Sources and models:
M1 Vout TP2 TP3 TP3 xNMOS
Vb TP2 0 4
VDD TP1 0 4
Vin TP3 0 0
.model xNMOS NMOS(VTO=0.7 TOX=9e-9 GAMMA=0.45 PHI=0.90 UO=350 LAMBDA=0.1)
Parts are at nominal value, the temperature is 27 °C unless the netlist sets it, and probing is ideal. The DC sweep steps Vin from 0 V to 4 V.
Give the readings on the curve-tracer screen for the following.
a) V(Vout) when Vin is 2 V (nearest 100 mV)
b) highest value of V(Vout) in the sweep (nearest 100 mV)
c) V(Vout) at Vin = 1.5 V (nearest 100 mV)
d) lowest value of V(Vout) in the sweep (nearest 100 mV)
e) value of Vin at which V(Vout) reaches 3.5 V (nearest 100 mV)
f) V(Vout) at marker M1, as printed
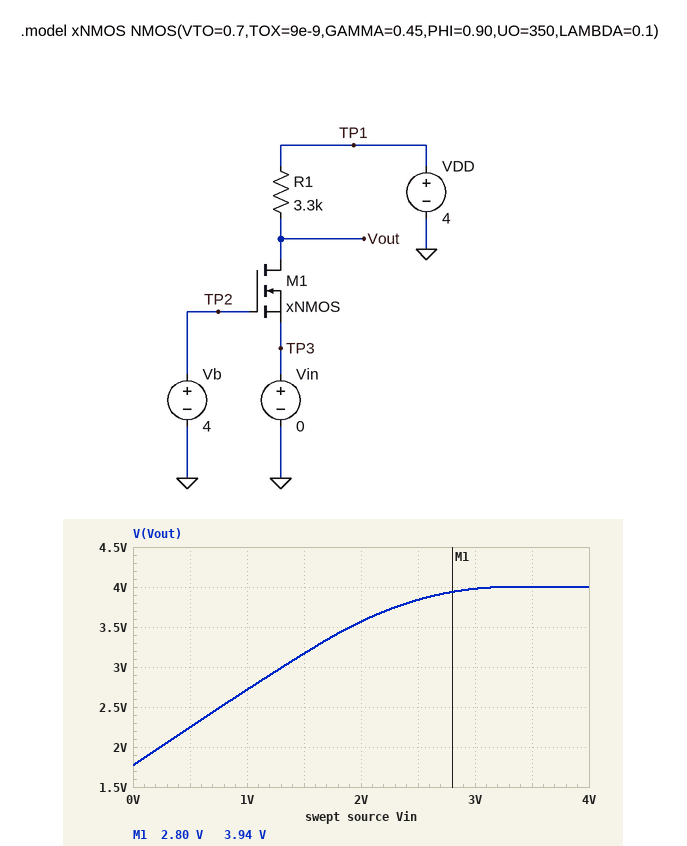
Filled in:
3.6 V
4.0 V
3.2 V
1.8 V
1.9 V
3.94 V
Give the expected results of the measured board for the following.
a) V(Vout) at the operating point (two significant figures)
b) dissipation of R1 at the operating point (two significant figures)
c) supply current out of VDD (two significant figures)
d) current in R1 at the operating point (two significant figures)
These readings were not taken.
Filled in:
1.8 V
1.5 mW
680 µA
680 µA
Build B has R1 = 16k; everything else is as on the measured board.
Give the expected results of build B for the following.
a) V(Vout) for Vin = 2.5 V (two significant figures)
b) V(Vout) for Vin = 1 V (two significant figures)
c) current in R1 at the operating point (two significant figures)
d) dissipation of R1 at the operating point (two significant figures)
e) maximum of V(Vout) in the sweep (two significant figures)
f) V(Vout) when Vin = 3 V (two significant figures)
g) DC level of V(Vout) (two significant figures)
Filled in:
3.3 V
1.5 V
220 µA
760 µW
4.0 V
3.9 V
510 mV
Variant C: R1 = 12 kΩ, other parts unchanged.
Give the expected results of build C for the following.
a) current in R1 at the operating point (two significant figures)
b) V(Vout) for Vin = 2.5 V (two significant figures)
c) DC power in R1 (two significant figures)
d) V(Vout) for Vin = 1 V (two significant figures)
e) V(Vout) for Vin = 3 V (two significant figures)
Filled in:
280 µA
3.4 V
930 µW
1.7 V
3.9 V
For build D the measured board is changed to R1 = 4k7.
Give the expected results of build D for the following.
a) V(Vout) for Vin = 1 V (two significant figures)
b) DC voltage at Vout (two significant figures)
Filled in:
2.4 V
1.4 V
